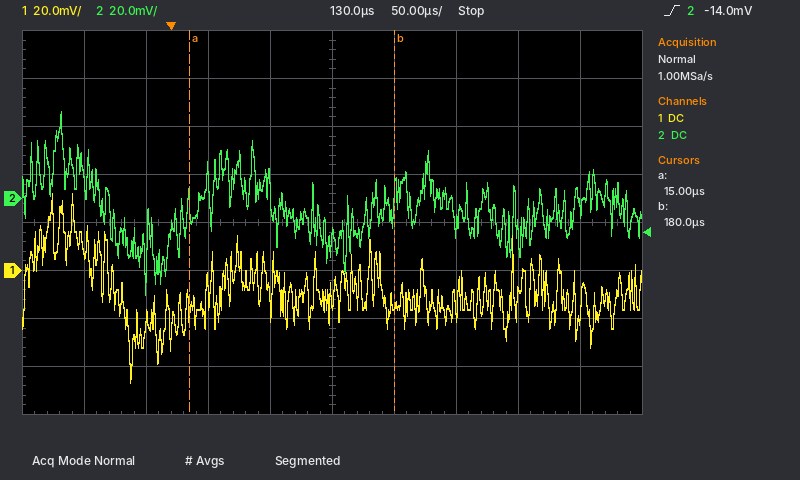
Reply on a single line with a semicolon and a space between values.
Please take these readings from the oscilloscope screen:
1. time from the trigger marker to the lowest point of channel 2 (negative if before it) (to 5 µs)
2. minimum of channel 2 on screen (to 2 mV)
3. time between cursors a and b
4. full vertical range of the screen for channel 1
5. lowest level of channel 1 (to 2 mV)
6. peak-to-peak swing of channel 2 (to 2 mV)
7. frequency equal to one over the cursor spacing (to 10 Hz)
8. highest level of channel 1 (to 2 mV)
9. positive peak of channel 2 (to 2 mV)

-20 µs; -40 mV; 165 µs; 160 mV; -46 mV; 76 mV; 6.06 kHz; 32 mV; 36 mV
